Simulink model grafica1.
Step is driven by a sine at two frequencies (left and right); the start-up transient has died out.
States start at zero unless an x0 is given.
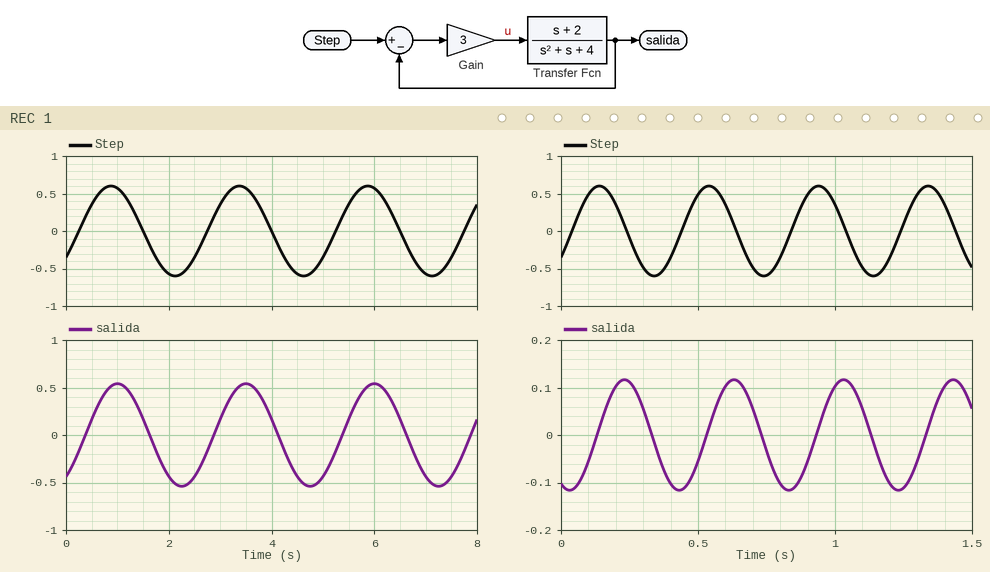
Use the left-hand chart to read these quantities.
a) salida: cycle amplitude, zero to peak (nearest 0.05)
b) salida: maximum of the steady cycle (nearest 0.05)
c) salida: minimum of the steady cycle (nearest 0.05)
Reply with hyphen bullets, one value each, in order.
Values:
- 0.55
- 0.55
- -0.55
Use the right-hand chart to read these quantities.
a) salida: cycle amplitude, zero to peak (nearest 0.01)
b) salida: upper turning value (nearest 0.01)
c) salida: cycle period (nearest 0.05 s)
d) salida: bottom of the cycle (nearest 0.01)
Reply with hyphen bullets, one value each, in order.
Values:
- 0.12
- 0.12
- 0.40 s
- -0.12
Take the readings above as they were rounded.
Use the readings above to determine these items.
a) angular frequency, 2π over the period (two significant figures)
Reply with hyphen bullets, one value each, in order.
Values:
- 16 rad/s
